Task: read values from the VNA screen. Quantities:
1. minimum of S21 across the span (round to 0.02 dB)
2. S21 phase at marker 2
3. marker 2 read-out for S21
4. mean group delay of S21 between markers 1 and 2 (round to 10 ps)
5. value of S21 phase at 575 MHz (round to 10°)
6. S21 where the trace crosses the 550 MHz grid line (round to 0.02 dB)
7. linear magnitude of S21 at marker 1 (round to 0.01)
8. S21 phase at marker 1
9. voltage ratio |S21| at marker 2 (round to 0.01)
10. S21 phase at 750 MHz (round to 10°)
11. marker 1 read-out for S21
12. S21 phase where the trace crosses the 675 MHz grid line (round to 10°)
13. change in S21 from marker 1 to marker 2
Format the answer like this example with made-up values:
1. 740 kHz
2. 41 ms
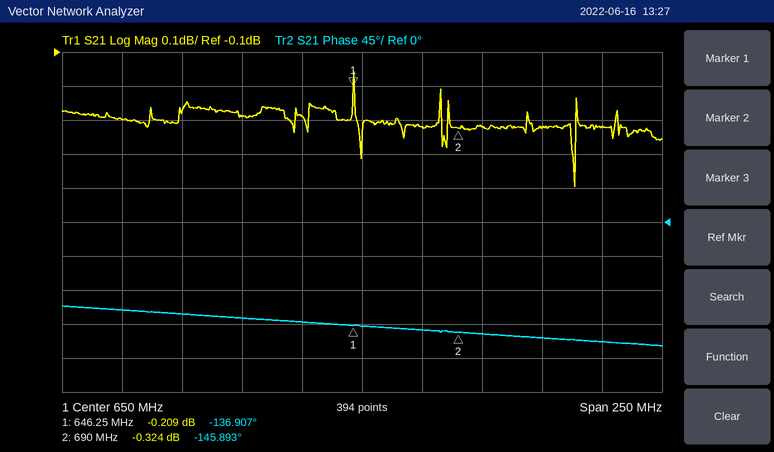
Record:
1. -0.50 dB
2. -145.893°
3. -0.324 dB
4. 570 ps
5. -120°
6. -0.30 dB
7. 0.98
8. -136.907°
9. 0.96
10. -160°
11. -0.209 dB
12. -140°
13. -0.115 dB
